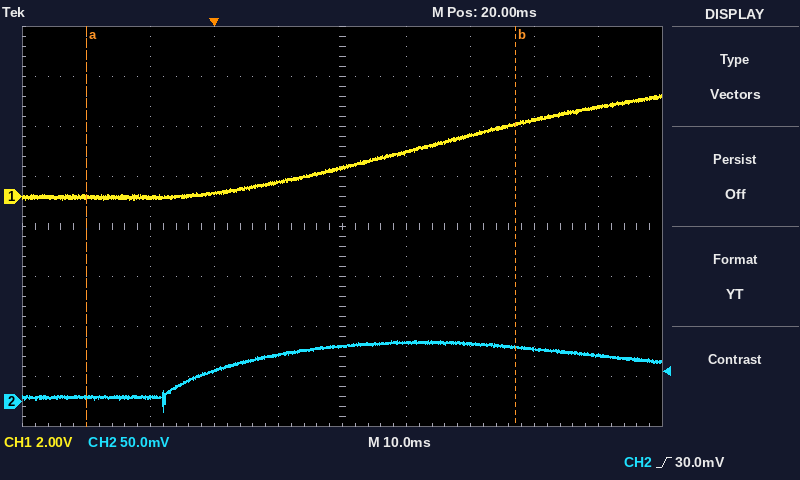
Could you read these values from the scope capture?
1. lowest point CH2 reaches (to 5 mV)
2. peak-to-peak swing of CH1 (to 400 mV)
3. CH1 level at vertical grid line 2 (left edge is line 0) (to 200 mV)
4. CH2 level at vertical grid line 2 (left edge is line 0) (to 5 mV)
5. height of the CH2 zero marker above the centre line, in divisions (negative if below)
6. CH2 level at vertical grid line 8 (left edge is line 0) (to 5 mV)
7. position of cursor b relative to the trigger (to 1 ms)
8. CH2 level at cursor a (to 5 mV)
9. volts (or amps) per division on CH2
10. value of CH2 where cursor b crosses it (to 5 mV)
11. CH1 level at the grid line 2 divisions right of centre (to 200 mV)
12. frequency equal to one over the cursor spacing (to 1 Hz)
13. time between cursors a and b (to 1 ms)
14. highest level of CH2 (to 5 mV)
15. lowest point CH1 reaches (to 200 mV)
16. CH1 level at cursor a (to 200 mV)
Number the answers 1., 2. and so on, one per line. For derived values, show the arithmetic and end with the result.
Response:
1. -10 mV
2. 4.4 V
3. 0.0 V
4. 5 mV
5. -3.5 div
6. 50 mV
7. +47 ms
8. 5 mV
9. 50 mV
10. 55 mV
11. 2.4 V
12. 1 / 67 ms ≈ 15 Hz
13. 67 ms
14. 60 mV
15. -200 mV
16. 0.0 V
